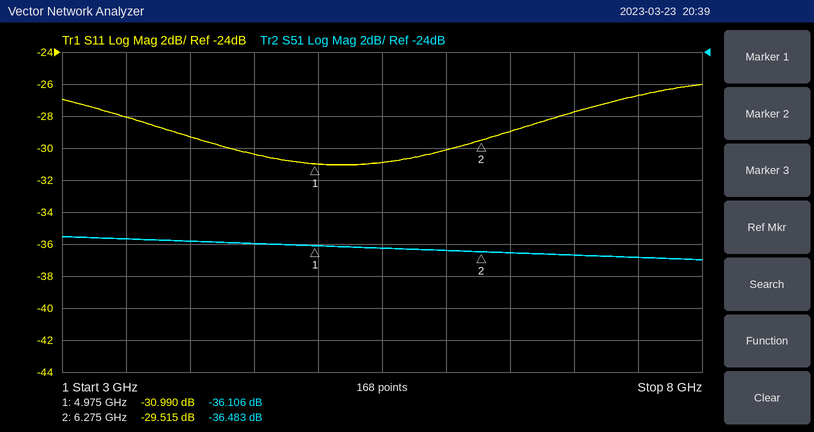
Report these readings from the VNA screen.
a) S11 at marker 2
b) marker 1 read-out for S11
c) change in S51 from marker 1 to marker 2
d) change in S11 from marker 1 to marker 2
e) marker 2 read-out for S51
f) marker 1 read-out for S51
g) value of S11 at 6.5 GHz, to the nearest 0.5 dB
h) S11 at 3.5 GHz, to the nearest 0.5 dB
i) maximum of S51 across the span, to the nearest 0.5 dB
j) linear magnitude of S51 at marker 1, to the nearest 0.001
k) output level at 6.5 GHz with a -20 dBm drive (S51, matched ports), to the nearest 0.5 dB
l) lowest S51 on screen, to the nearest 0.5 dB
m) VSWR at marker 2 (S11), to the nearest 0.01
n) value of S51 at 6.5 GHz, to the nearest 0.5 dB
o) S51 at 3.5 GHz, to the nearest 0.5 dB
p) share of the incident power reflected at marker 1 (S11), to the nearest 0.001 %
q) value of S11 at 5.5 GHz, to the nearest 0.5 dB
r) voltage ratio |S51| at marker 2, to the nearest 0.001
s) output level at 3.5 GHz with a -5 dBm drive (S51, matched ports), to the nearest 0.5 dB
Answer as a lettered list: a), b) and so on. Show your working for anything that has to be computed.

a) -29.515 dB
b) -30.990 dB
c) -36.483 − (-36.106) = -0.377 dB
d) -29.515 − (-30.99) = 1.475 dB
e) -36.483 dB
f) -36.106 dB
g) -29.0 dB
h) -28.0 dB
i) -35.5 dB
j) 10^(-36.106/20) ≈ 0.016
k) -20 dBm + (-36.5 dB) = -56.5 dBm
l) -37.0 dB
m) (1 + 0.0334)/(1 − 0.0334) ≈ 1.07
n) -36.5 dB
o) -35.5 dB
p) 10^(-30.99/10) ≈ 0.080 %
q) -31.0 dB
r) 10^(-36.483/20) ≈ 0.015
s) -5 dBm + (-35.5 dB) = -40.5 dBm
